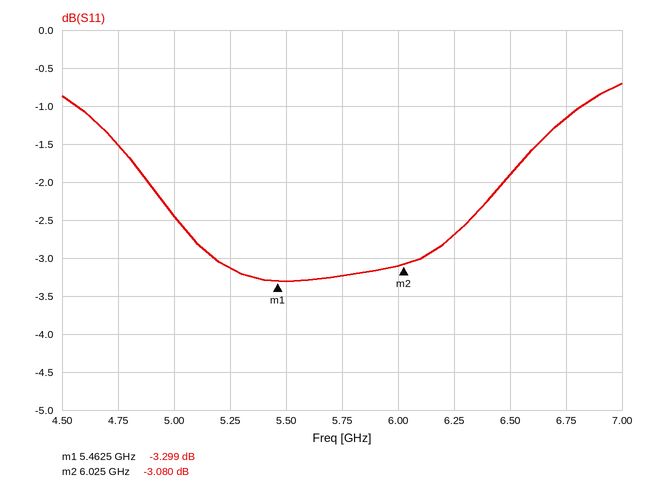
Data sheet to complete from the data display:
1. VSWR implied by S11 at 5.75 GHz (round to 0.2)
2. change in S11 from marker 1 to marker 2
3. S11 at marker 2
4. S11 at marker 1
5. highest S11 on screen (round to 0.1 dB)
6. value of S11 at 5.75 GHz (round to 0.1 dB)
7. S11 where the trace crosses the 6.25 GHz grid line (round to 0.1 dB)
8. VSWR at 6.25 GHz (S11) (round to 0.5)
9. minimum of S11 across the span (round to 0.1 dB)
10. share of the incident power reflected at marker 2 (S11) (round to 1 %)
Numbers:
5.4
0.219 dB
-3.080 dB
-3.299 dB
-0.7 dB
-3.2 dB
-2.7 dB
6.5
-3.3 dB
49 %
